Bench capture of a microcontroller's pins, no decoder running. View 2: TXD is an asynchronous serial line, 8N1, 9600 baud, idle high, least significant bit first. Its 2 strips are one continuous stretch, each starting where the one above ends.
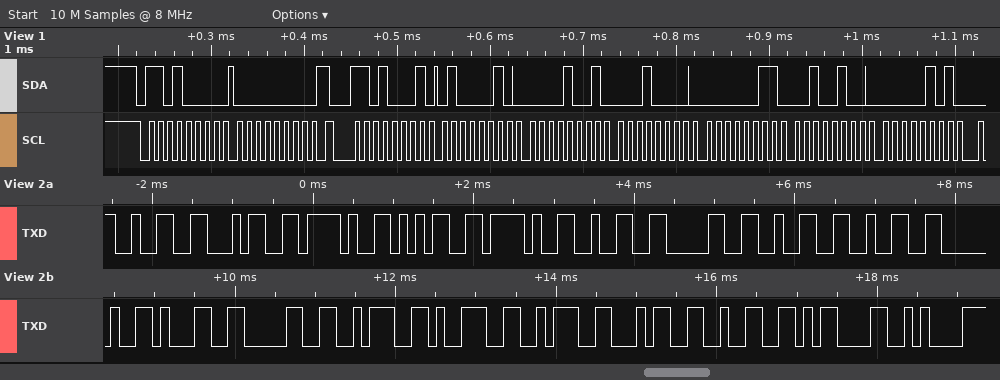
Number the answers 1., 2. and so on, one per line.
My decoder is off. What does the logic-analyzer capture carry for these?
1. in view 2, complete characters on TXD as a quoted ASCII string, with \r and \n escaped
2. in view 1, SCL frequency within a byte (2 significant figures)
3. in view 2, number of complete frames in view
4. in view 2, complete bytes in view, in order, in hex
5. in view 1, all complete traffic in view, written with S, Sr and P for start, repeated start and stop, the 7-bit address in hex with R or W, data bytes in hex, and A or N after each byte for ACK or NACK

1. "24/5/2022 10:9:42\r\n"
2. 100 kHz
3. 19
4. 32 34 2F 35 2F 32 30 32 32 20 31 30 3A 39 3A 34 32 0D 0A
5. S 68W A 00 A Sr 68R A 42 A 09 A 10 A 03 A 24 A 05 A
